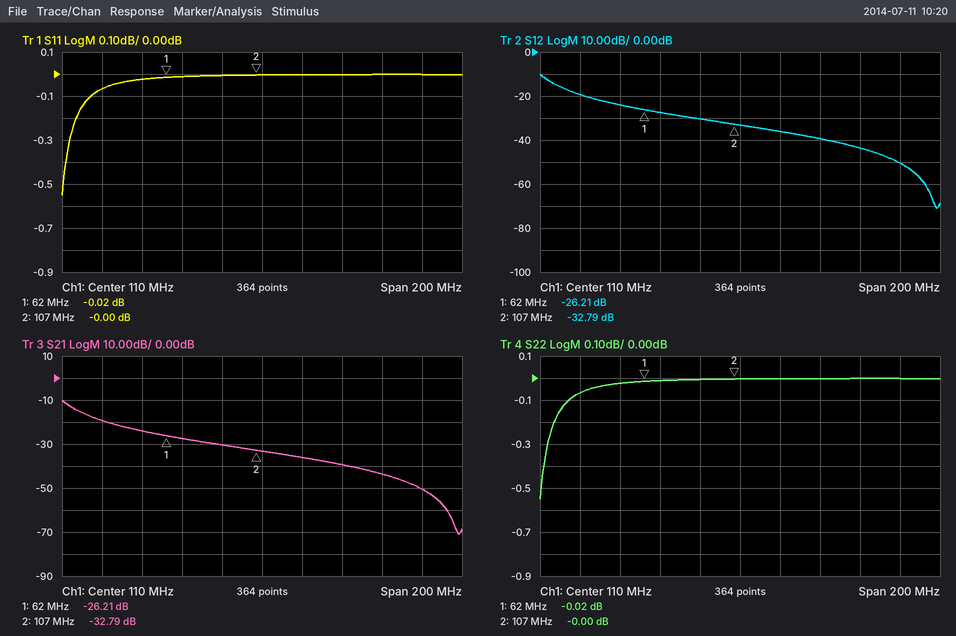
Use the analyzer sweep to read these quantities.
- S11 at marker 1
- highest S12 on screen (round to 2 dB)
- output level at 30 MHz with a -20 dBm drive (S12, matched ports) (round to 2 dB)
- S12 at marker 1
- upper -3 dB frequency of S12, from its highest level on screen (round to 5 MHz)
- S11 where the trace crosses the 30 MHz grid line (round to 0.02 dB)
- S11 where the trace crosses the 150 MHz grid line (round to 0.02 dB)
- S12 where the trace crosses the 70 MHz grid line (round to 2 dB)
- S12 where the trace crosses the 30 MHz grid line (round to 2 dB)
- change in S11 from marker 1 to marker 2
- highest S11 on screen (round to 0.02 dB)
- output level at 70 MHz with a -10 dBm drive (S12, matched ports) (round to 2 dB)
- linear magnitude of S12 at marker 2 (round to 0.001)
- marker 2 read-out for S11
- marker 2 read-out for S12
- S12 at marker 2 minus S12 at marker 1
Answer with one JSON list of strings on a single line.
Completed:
["-0.02 dB", "-10 dB", "-40 dBm", "-26.21 dB", "15 MHz", "-0.06 dB", "0.00 dB", "-28 dB", "-20 dB", "0.02 dB", "0.00 dB", "-38 dBm", "0.023", "-0.00 dB", "-32.79 dB", "-6.58 dB"]
